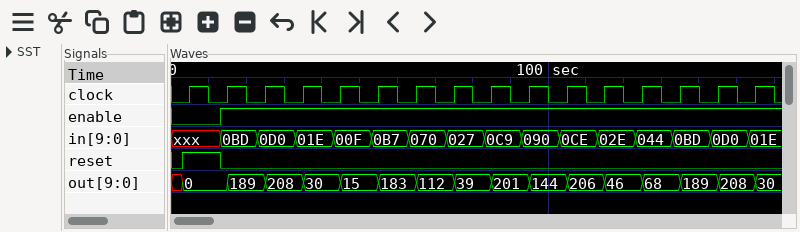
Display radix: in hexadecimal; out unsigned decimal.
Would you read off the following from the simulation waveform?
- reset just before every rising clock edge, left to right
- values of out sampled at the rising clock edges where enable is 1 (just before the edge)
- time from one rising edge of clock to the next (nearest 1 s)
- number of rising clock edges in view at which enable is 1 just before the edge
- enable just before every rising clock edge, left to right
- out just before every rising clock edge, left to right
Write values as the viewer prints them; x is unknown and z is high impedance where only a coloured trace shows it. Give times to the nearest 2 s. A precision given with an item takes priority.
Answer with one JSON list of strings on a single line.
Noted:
["1 0 0 0 0 0 0 0 0 0 0 0 0 0 0 0", "0, 189, 208, 30, 15, 183, 112, 39, 201, 144, 206, 46, 68, 189, 208", "10 s", "15", "0 1 1 1 1 1 1 1 1 1 1 1 1 1 1 1", "0, 0, 189, 208, 30, 15, 183, 112, 39, 201, 144, 206, 46, 68, 189, 208"]
